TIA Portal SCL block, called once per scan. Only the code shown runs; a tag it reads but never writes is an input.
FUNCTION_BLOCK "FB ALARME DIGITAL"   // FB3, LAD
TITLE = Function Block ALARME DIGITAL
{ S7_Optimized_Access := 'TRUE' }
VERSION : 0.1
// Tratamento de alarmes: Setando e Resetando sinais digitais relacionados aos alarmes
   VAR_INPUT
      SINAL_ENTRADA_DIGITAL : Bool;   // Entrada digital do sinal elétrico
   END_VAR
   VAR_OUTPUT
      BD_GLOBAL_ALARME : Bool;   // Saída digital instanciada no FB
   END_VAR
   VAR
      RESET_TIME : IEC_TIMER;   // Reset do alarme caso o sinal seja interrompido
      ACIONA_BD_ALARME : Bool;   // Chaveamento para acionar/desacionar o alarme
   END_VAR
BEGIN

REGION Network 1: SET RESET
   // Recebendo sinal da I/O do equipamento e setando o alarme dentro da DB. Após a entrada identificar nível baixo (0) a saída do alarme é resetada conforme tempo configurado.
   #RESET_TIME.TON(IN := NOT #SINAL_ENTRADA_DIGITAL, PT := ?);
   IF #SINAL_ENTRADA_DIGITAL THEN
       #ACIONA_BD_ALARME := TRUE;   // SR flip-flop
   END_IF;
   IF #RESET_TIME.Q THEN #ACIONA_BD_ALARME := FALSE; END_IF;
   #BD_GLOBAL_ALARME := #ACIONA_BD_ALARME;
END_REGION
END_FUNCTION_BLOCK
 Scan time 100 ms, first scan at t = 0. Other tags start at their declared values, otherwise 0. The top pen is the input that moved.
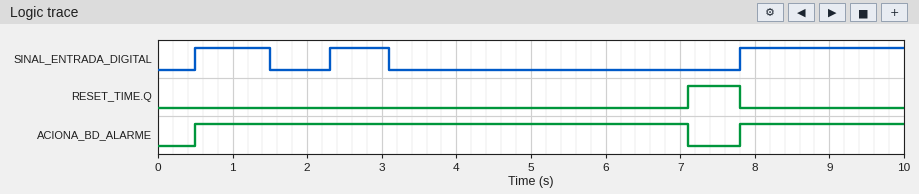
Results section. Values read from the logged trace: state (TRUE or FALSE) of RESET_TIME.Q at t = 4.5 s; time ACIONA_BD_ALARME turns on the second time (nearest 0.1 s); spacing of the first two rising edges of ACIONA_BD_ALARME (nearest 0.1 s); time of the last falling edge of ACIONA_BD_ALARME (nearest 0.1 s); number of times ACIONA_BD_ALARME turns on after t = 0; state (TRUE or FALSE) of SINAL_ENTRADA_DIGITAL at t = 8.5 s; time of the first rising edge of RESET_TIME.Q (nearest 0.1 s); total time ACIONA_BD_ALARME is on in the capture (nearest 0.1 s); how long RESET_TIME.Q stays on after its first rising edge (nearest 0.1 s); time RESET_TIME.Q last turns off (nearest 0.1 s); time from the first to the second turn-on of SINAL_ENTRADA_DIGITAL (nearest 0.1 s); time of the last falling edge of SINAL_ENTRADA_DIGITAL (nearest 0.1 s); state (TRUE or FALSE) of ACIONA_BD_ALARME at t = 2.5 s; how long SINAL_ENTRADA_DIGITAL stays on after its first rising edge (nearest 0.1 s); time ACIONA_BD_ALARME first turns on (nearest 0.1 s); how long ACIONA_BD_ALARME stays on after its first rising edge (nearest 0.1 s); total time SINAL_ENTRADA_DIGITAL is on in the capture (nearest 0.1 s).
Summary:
FALSE
7.8 s
7.3 s
7.1 s
2
TRUE
7.1 s
8.8 s
0.7 s
7.8 s
1.8 s
3.1 s
TRUE
1.0 s
0.5 s
6.6 s
4.0 s
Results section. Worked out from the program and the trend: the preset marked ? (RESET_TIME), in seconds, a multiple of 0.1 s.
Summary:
4.0 s
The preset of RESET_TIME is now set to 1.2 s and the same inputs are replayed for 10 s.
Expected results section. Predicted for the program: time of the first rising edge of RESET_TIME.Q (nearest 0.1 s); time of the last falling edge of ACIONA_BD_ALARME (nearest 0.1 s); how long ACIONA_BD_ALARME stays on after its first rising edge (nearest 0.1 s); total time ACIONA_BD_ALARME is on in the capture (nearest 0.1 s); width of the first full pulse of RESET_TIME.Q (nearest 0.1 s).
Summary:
4.3 s
4.3 s
3.8 s
6.0 s
3.5 s
